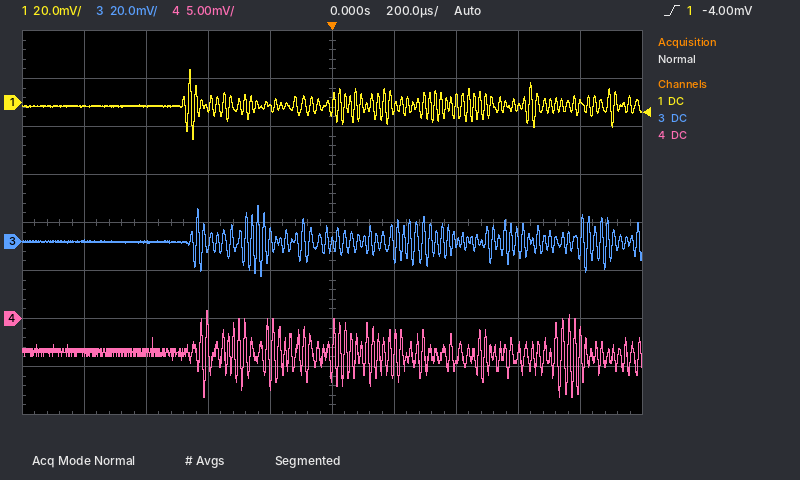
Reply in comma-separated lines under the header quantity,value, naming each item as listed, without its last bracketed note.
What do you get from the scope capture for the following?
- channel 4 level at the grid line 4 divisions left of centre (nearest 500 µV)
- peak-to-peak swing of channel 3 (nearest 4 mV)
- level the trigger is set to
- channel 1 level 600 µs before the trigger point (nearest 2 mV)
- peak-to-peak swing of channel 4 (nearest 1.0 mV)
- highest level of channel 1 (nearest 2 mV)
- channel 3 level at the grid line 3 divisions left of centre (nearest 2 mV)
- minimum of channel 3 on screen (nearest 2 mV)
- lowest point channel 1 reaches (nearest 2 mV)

quantity,value
channel 4 level at the grid line 4 divisions left of centre,-3.5 mV
peak-to-peak swing of channel 3,28 mV
level the trigger is set to,-4.00 mV
channel 1 level 600 µs before the trigger point,-2 mV
peak-to-peak swing of channel 4,9.0 mV
highest level of channel 1,14 mV
channel 3 level at the grid line 3 divisions left of centre,0 mV
minimum of channel 3 on screen,-14 mV
lowest point channel 1 reaches,-16 mV
